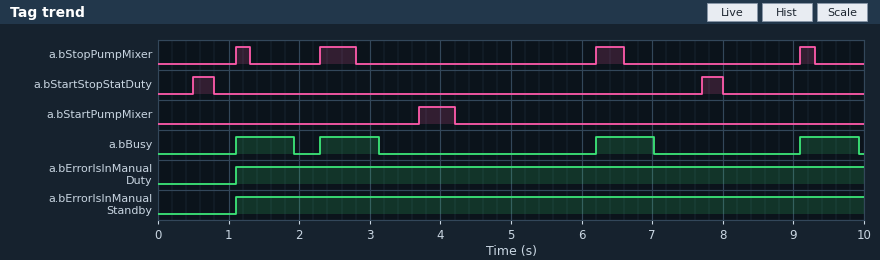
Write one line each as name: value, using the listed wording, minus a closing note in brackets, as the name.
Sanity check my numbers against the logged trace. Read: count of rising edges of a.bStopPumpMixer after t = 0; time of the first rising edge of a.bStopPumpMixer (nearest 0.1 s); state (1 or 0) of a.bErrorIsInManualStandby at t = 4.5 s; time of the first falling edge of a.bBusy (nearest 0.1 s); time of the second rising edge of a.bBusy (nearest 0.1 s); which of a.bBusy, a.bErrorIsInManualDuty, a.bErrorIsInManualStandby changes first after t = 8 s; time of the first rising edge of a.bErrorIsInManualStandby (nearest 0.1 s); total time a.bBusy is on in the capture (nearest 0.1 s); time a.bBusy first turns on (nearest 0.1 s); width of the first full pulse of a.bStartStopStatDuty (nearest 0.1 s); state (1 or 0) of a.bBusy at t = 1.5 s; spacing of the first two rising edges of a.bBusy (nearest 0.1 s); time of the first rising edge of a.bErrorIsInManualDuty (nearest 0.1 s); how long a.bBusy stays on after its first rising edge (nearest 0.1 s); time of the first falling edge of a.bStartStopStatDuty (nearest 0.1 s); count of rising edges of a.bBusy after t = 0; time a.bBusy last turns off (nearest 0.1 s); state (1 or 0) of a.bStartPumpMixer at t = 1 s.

count of rising edges of a.bStopPumpMixer after t = 0: 4
time of the first rising edge of a.bStopPumpMixer: 1.1 s
state (1 or 0) of a.bErrorIsInManualStandby at t = 4.5 s: 1
time of the first falling edge of a.bBusy: 1.9 s
time of the second rising edge of a.bBusy: 2.3 s
which of a.bBusy, a.bErrorIsInManualDuty, a.bErrorIsInManualStandby changes first after t = 8 s: a.bBusy
time of the first rising edge of a.bErrorIsInManualStandby: 1.1 s
total time a.bBusy is on in the capture: 3.3 s
time a.bBusy first turns on: 1.1 s
width of the first full pulse of a.bStartStopStatDuty: 0.3 s
state (1 or 0) of a.bBusy at t = 1.5 s: 1
spacing of the first two rising edges of a.bBusy: 1.2 s
time of the first rising edge of a.bErrorIsInManualDuty: 1.1 s
how long a.bBusy stays on after its first rising edge: 0.8 s
time of the first falling edge of a.bStartStopStatDuty: 0.8 s
count of rising edges of a.bBusy after t = 0: 4
time a.bBusy last turns off: 9.9 s
state (1 or 0) of a.bStartPumpMixer at t = 1 s: 0
